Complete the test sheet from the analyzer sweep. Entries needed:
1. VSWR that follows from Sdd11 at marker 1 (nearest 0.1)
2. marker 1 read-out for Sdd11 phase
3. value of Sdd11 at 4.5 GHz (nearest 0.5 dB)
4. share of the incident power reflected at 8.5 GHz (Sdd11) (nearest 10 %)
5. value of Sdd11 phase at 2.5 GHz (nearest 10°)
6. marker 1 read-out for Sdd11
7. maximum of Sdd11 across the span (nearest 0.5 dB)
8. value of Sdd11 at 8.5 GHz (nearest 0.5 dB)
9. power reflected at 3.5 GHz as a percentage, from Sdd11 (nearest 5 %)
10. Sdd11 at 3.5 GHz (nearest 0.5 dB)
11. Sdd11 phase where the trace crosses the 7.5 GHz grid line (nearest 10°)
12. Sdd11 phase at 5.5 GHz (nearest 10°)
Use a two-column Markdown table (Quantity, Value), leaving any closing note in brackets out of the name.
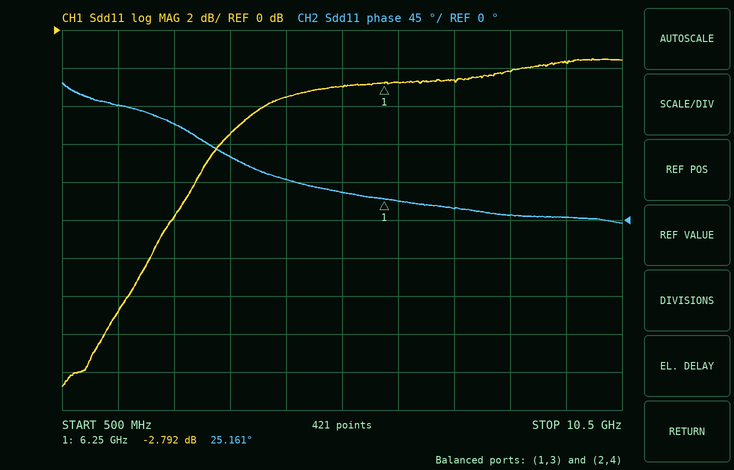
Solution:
| Quantity | Value |
|---|---|
| VSWR that follows from Sdd11 at marker 1 | 6.3 |
| marker 1 read-out for Sdd11 phase | 25.161° |
| value of Sdd11 at 4.5 GHz | -3.5 dB |
| share of the incident power reflected at 8.5 GHz (Sdd11) | 60 % |
| value of Sdd11 phase at 2.5 GHz | 110° |
| marker 1 read-out for Sdd11 | -2.792 dB |
| maximum of Sdd11 across the span | -1.5 dB |
| value of Sdd11 at 8.5 GHz | -2.0 dB |
| power reflected at 3.5 GHz as a percentage, from Sdd11 | 30 % |
| Sdd11 at 3.5 GHz | -5.5 dB |
| Sdd11 phase where the trace crosses the 7.5 GHz grid line | 10° |
| Sdd11 phase at 5.5 GHz | 30° |
